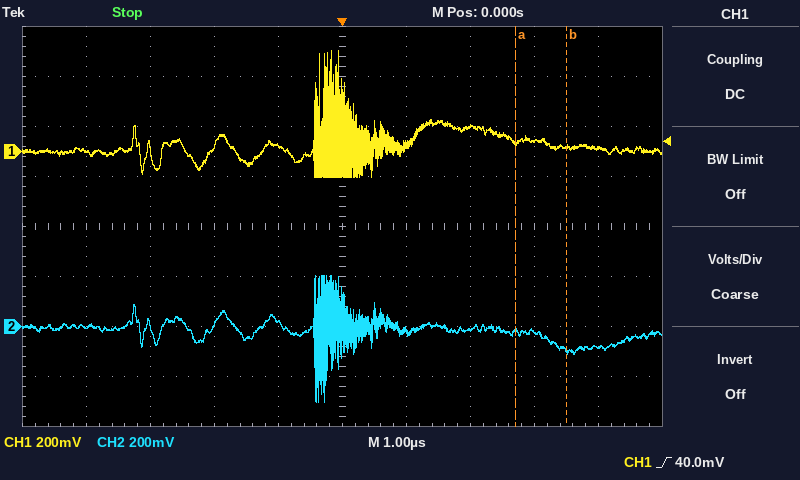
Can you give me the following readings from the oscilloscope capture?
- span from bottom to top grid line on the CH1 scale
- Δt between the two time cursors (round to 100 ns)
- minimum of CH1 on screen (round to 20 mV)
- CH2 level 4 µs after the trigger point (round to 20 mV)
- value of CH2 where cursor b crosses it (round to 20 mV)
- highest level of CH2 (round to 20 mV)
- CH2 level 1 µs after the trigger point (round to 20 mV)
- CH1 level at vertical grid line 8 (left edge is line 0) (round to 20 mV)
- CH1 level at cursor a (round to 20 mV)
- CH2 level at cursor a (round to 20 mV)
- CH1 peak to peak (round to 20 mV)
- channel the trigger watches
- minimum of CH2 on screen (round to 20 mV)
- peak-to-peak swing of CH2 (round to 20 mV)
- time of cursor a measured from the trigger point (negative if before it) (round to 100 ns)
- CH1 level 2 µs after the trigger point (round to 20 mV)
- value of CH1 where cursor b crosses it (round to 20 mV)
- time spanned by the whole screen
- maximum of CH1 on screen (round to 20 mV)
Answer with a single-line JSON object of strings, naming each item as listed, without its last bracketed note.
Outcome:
{"span from bottom to top grid line on the CH1 scale": "1.6 V", "Δt between the two time cursors": "800 ns", "minimum of CH1 on screen": "-100 mV", "CH2 level 4 µs after the trigger point": "-80 mV", "value of CH2 where cursor b crosses it": "-100 mV", "highest level of CH2": "200 mV", "CH2 level 1 µs after the trigger point": "-20 mV", "CH1 level at vertical grid line 8 (left edge is line 0)": "40 mV", "CH1 level at cursor a": "40 mV", "CH2 level at cursor a": "-20 mV", "CH1 peak to peak": "500 mV", "channel the trigger watches": "CH1", "minimum of CH2 on screen": "-300 mV", "peak-to-peak swing of CH2": "500 mV", "time of cursor a measured from the trigger point (negative if before it)": "+2.7 µs", "CH1 level 2 µs after the trigger point": "100 mV", "value of CH1 where cursor b crosses it": "20 mV", "time spanned by the whole screen": "10 µs", "maximum of CH1 on screen": "400 mV"}
